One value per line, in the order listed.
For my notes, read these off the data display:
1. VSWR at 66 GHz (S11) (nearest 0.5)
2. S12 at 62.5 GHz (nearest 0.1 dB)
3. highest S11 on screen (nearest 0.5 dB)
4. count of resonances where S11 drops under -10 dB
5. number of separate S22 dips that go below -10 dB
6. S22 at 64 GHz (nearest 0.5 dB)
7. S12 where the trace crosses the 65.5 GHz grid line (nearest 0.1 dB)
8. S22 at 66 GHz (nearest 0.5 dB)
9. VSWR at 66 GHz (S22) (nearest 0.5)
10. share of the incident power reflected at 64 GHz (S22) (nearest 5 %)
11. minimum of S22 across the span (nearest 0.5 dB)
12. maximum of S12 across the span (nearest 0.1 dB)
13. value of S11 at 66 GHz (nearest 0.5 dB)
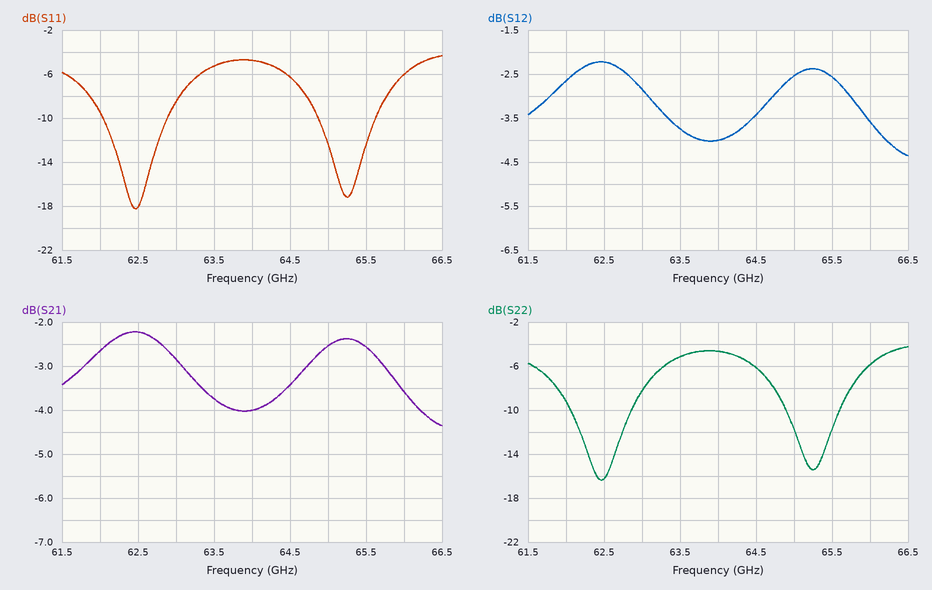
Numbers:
3.0
-2.2 dB
-4.5 dB
2
2
-4.5 dB
-2.6 dB
-6.0 dB
3.0
35 %
-16.5 dB
-2.2 dB
-6.0 dB
